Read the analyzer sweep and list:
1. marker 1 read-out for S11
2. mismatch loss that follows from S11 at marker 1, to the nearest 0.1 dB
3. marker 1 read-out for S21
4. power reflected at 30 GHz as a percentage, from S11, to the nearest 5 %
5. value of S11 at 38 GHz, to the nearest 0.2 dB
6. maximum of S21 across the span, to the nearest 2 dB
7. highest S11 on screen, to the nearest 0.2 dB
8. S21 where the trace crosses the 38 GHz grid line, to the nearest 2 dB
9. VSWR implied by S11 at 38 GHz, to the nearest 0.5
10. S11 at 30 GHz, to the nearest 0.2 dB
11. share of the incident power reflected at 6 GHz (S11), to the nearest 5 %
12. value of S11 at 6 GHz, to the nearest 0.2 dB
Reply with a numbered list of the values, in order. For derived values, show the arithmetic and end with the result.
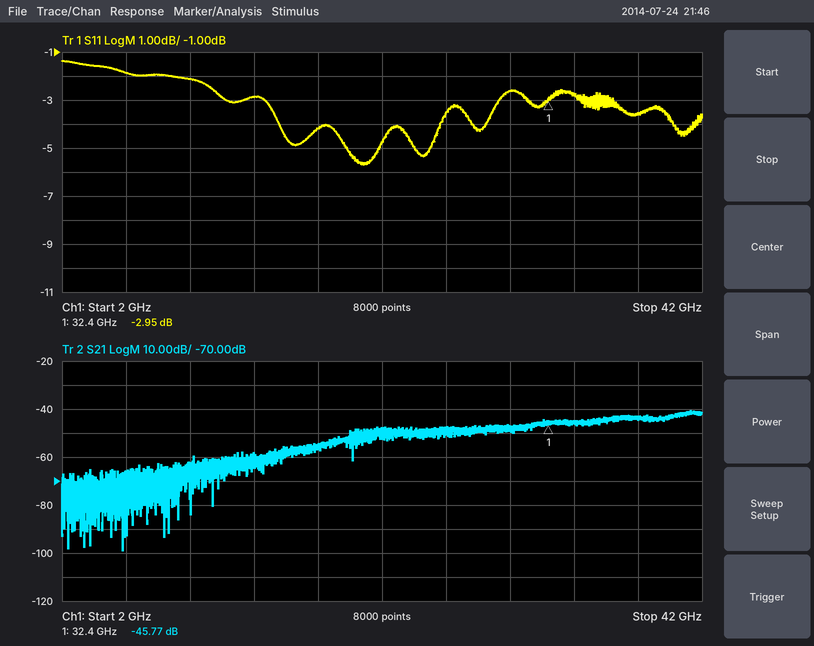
1. -2.95 dB
2. −10 log10(1 − 10^(-2.95/10)) ≈ 3.1 dB
3. -45.77 dB
4. 10^(-2.6/10) ≈ 55 %
5. -3.6 dB
6. -40 dB
7. -1.4 dB
8. -44 dB
9. |Γ| = 10^(-3.6/20) = 0.6607; VSWR = (1 + 0.6607)/(1 − 0.6607) ≈ 4.89, so 5.0 to the nearest 0.5
10. -2.6 dB
11. 10^(-1.8/10) ≈ 66.1 %, so 65 % to the nearest 5 %
12. -1.8 dB
